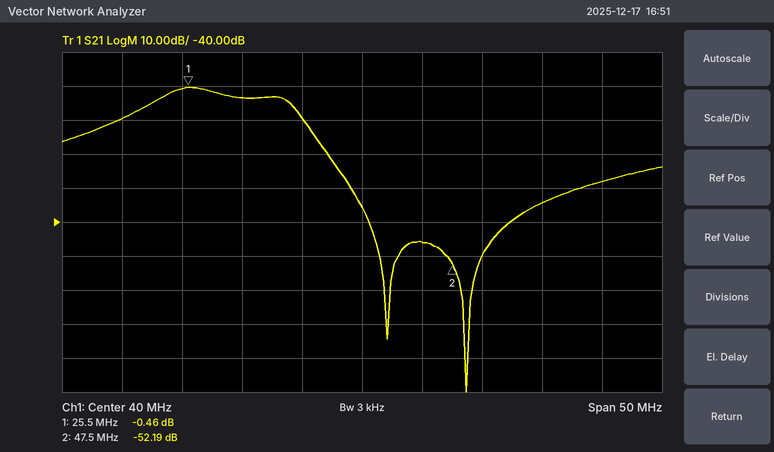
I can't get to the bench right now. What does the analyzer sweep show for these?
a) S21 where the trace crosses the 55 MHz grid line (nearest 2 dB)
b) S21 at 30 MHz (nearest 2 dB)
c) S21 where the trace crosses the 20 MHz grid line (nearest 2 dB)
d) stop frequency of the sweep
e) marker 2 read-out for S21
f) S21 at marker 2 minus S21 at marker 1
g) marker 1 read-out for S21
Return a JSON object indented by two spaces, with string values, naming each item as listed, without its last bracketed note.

{
  "S21 where the trace crosses the 55 MHz grid line": "-34 dB",
  "S21 at 30 MHz": "-4 dB",
  "S21 where the trace crosses the 20 MHz grid line": "-10 dB",
  "stop frequency of the sweep": "65 MHz",
  "marker 2 read-out for S21": "-52.19 dB",
  "S21 at marker 2 minus S21 at marker 1": "-51.73 dB",
  "marker 1 read-out for S21": "-0.46 dB"
}
